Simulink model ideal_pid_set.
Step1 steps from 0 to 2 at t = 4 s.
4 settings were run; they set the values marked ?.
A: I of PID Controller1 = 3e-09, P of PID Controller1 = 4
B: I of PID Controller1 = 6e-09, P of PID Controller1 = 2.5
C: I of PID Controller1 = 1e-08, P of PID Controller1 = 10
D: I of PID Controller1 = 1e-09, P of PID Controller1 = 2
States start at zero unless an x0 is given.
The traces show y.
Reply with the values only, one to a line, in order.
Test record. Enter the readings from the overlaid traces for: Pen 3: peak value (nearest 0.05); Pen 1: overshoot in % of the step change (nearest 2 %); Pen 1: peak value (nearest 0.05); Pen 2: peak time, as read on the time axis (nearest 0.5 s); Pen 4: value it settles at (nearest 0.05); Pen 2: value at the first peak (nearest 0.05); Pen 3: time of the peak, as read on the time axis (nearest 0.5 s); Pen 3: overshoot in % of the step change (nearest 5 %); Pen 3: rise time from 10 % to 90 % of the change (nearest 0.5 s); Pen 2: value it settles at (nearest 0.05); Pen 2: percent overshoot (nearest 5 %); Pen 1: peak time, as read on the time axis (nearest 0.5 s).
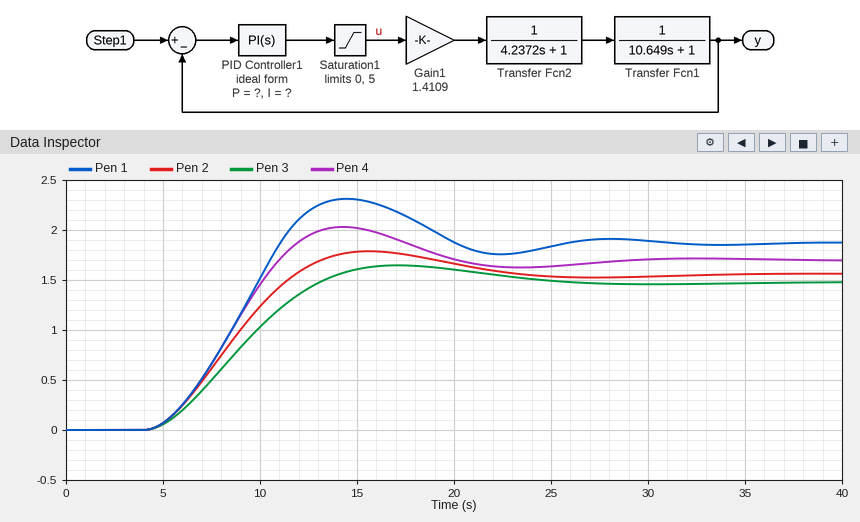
1.65
24 %
2.30
15.5 s
1.70
1.80
17.0 s
10 %
6.0 s
1.55
15 %
14.5 s
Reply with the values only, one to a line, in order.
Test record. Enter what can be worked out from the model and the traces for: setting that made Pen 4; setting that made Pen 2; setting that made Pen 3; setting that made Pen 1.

A
B
D
C
